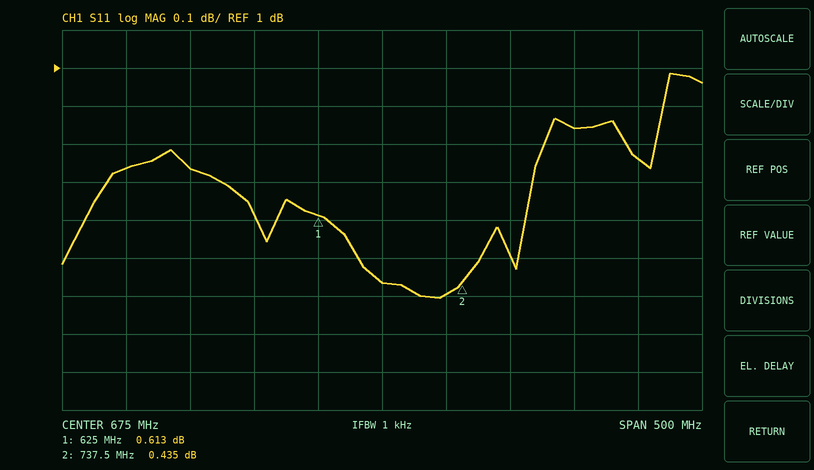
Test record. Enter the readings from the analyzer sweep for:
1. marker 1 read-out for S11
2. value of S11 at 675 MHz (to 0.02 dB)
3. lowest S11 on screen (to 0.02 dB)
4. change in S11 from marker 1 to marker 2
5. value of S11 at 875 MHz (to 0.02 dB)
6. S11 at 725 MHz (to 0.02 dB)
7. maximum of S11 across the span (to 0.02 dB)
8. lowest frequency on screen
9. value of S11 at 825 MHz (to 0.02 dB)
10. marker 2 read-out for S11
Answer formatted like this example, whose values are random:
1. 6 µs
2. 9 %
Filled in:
1. 0.613 dB
2. 0.44 dB
3. 0.40 dB
4. -0.178 dB
5. 0.76 dB
6. 0.40 dB
7. 0.98 dB
8. 425 MHz
9. 0.84 dB
10. 0.435 dB
